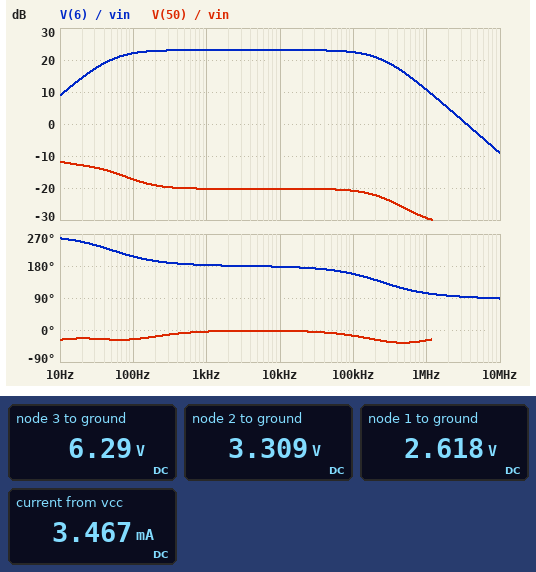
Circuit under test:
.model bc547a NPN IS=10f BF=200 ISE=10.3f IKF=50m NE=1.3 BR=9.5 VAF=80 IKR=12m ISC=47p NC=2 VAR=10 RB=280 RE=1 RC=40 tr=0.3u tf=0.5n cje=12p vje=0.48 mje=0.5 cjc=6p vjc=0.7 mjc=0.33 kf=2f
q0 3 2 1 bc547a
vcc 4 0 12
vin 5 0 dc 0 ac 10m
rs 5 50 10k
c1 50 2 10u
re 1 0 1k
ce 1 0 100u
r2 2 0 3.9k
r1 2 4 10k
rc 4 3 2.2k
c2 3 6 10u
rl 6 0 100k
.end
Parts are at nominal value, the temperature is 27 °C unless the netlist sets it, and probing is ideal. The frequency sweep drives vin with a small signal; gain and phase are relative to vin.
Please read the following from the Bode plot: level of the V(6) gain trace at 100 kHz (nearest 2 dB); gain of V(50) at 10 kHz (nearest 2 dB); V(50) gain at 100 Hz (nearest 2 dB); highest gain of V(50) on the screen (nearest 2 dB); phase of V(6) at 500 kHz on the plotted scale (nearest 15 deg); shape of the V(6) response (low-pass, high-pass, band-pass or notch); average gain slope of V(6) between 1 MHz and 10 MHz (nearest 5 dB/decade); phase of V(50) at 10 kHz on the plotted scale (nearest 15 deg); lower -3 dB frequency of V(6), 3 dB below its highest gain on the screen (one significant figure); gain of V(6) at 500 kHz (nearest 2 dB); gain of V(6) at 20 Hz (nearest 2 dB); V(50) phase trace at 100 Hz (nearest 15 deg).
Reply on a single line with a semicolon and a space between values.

22 dB; -20 dB; -18 dB; -12 dB; 120 deg; band-pass; -20 dB/decade; 0 deg; 50 Hz; 16 dB; 14 dB; -30 deg
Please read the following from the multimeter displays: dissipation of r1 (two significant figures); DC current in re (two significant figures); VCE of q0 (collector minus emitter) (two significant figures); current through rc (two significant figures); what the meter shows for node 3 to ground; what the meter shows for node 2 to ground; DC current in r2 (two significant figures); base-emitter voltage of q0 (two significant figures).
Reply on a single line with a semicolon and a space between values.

7.6 mW; 2.6 mA; 3.7 V; 2.6 mA; 6.29 V; 3.309 V; 850 µA; 690 mV
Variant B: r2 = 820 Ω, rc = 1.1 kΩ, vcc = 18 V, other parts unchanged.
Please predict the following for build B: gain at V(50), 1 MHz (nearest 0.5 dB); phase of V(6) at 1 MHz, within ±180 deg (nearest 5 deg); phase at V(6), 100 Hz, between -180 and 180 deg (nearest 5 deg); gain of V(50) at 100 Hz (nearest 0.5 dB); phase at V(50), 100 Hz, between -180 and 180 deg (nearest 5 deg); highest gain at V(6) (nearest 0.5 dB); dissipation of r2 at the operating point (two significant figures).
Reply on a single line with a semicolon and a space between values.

-25.0 dB; 150 deg; -160 deg; -23.5 dB; -15 deg; 4.5 dB; 2.3 mW
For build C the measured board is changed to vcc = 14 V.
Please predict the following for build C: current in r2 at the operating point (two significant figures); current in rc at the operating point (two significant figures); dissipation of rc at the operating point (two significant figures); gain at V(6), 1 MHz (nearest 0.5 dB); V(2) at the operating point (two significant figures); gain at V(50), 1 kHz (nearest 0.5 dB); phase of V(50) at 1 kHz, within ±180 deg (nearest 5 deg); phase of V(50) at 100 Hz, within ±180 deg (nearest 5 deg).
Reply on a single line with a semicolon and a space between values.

990 µA; 3.1 mA; 22 mW; 11.0 dB; 3.9 V; -21.0 dB; -5 deg; -30 deg
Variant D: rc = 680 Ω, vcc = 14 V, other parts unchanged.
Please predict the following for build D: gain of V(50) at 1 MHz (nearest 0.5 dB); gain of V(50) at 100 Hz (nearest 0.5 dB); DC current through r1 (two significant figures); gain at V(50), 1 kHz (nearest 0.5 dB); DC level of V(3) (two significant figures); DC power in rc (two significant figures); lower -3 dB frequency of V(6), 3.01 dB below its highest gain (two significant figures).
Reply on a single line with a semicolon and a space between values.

-25.0 dB; -17.0 dB; 1.0 mA; -20.5 dB; 12 V; 6.7 mW; 58 Hz
